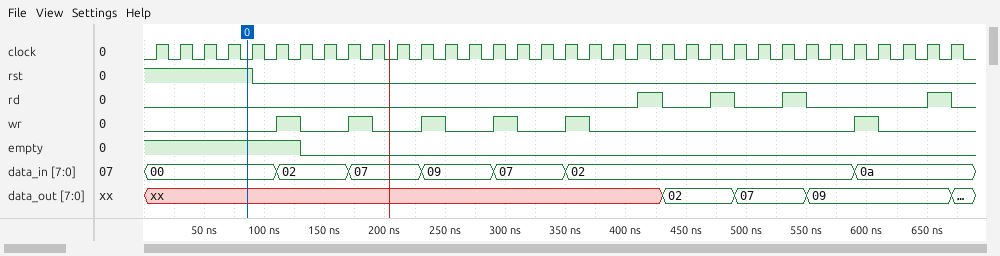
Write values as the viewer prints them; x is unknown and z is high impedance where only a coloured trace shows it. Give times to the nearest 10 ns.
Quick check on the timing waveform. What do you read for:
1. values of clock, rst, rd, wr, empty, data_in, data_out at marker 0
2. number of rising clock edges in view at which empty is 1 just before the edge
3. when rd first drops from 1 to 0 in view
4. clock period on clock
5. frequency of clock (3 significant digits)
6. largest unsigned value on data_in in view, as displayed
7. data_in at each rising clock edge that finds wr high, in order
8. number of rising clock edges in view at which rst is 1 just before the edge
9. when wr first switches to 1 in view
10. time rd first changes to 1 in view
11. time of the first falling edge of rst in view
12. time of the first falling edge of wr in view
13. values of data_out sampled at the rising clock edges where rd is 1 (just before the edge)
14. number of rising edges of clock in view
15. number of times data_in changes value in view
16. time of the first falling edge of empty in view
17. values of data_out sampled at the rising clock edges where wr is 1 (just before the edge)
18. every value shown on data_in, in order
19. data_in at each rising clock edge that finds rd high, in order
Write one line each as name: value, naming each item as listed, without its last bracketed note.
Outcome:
values of clock, rst, rd, wr, empty, data_in, data_out at marker 0: clock=0, rst=1, rd=0, wr=0, empty=1, data_in=00, data_out=xx
number of rising clock edges in view at which empty is 1 just before the edge: 7
when rd first drops from 1 to 0 in view: 430 ns
clock period on clock: 20 ns
frequency of clock: 50.0 MHz
largest unsigned value on data_in in view, as displayed: 0a
data_in at each rising clock edge that finds wr high, in order: 02, 07, 09, 07, 02, 0a
number of rising clock edges in view at which rst is 1 just before the edge: 5
when wr first switches to 1 in view: 110 ns
time rd first changes to 1 in view: 410 ns
time of the first falling edge of rst in view: 90 ns
time of the first falling edge of wr in view: 130 ns
values of data_out sampled at the rising clock edges where rd is 1: xx, 02, 07, 09
number of rising edges of clock in view: 34
number of times data_in changes value in view: 6
time of the first falling edge of empty in view: 130 ns
values of data_out sampled at the rising clock edges where wr is 1: xx, xx, xx, xx, xx, 09
every value shown on data_in, in order: 00, 02, 07, 09, 07, 02, 0a
data_in at each rising clock edge that finds rd high, in order: 02, 02, 02, 0a
